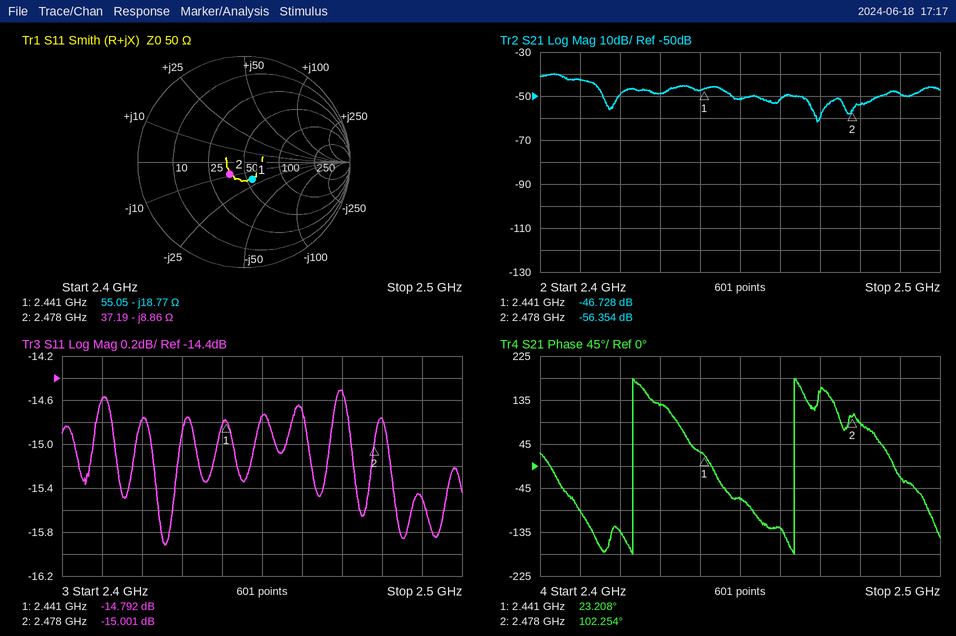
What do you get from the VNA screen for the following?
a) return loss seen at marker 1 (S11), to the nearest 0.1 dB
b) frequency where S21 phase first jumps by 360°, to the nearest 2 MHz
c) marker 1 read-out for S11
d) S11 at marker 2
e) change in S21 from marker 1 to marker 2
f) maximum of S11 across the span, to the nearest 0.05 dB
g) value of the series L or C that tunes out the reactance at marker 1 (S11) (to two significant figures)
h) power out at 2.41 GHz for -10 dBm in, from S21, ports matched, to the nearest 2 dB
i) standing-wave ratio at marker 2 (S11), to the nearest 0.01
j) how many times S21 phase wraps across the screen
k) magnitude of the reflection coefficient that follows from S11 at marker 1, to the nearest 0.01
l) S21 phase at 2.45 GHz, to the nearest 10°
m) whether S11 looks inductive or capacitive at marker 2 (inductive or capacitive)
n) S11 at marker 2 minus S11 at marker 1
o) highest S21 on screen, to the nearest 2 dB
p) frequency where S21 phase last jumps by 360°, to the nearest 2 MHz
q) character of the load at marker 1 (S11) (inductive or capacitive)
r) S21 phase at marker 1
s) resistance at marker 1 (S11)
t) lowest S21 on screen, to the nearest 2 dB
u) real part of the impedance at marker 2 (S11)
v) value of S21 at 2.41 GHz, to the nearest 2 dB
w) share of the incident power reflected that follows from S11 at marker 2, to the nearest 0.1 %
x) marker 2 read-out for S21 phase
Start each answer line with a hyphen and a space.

- 14.8 dB
- 2.424 GHz
- -14.792 dB
- -15.001 dB
- -9.626 dB
- -14.50 dB
- 1.2 nH
- -52 dBm
- 1.43
- 2
- 0.18
- -70°
- capacitive
- -0.209 dB
- -40 dB
- 2.464 GHz
- capacitive
- 23.208°
- 55.05 Ω
- -62 dB
- 37.19 Ω
- -42 dB
- 3.2 %
- 102.254°
